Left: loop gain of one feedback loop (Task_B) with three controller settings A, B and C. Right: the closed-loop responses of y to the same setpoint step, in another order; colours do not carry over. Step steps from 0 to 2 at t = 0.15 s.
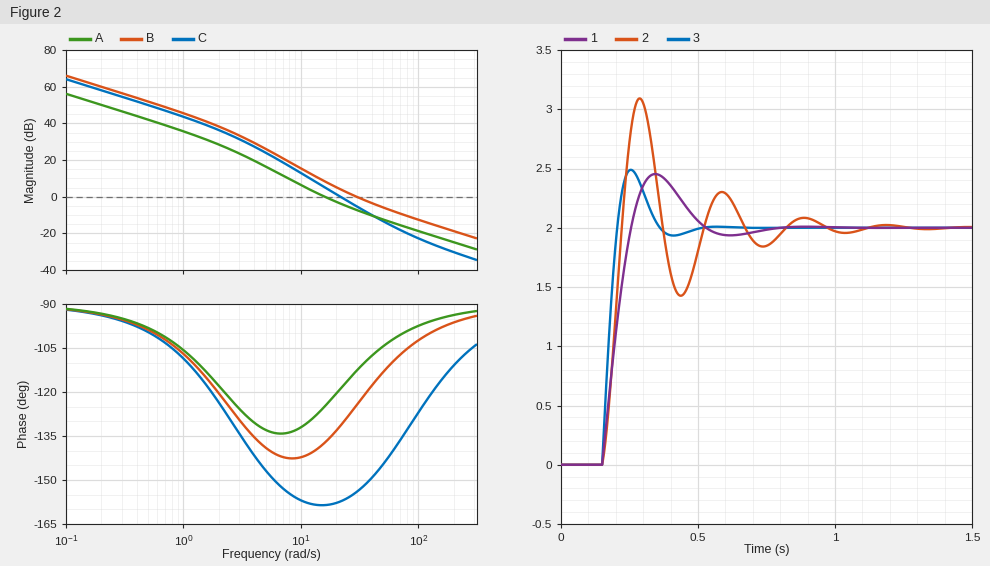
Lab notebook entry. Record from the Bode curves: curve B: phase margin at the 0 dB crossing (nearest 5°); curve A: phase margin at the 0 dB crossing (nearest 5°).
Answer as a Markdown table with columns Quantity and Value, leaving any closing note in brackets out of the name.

| Quantity | Value |
|---|---|
| curve B: phase margin at the 0 dB crossing | 55° |
| curve A: phase margin at the 0 dB crossing | 55° |
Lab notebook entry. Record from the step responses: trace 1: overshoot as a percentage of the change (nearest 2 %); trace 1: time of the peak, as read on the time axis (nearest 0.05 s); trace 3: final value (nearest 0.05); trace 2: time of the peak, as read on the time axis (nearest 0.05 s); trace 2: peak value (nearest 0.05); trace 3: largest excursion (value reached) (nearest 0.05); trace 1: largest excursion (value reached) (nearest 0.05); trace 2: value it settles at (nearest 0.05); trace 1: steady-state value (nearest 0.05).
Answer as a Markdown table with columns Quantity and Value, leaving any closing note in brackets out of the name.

| Quantity | Value |
|---|---|
| trace 1: overshoot as a percentage of the change | 22 % |
| trace 1: time of the peak, as read on the time axis | 0.35 s |
| trace 3: final value | 2.00 |
| trace 2: time of the peak, as read on the time axis | 0.30 s |
| trace 2: peak value | 3.10 |
| trace 3: largest excursion (value reached) | 2.50 |
| trace 1: largest excursion (value reached) | 2.45 |
| trace 2: value it settles at | 2.00 |
| trace 1: steady-state value | 2.00 |
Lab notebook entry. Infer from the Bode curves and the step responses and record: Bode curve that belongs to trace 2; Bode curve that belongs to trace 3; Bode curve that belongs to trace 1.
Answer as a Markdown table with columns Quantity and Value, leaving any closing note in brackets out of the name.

| Quantity | Value |
|---|---|
| Bode curve that belongs to trace 2 | C |
| Bode curve that belongs to trace 3 | B |
| Bode curve that belongs to trace 1 | A |
